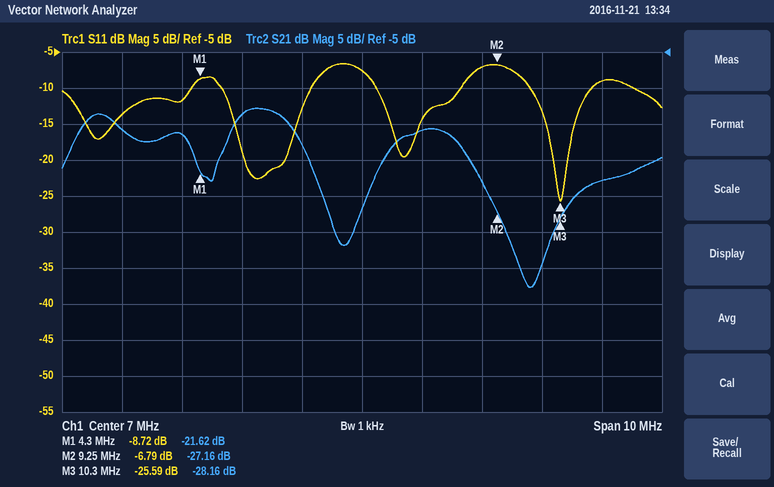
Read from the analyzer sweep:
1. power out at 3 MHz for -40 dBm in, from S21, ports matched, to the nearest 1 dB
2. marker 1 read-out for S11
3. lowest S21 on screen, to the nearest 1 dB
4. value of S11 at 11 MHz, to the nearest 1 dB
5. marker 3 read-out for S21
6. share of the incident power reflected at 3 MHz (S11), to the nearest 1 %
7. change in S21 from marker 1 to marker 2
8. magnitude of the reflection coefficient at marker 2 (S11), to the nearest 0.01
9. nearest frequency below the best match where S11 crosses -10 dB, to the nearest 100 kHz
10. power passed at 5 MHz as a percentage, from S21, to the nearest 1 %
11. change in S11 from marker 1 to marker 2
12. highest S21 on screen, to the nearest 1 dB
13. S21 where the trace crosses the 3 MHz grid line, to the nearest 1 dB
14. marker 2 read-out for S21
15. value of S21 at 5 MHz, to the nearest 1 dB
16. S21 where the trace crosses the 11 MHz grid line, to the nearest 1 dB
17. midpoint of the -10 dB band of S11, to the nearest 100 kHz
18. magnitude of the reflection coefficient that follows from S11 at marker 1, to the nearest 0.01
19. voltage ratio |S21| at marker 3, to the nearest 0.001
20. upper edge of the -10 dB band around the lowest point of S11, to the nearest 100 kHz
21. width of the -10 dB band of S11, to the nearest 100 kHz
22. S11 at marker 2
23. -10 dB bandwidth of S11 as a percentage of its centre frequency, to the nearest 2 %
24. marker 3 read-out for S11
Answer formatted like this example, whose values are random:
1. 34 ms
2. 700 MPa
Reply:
1. -56 dBm
2. -8.72 dB
3. -38 dB
4. -9 dB
5. -28.16 dB
6. 4 %
7. -5.54 dB
8. 0.46
9. 9.8 MHz
10. 4 %
11. 1.93 dB
12. -13 dB
13. -16 dB
14. -27.16 dB
15. -14 dB
16. -23 dB
17. 10.3 MHz
18. 0.37
19. 0.039
20. 10.8 MHz
21. 1.0 MHz
22. -6.79 dB
23. 10 %
24. -25.59 dB
